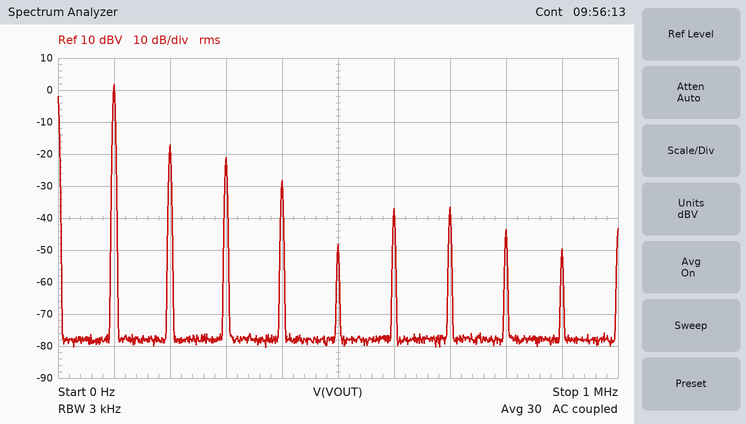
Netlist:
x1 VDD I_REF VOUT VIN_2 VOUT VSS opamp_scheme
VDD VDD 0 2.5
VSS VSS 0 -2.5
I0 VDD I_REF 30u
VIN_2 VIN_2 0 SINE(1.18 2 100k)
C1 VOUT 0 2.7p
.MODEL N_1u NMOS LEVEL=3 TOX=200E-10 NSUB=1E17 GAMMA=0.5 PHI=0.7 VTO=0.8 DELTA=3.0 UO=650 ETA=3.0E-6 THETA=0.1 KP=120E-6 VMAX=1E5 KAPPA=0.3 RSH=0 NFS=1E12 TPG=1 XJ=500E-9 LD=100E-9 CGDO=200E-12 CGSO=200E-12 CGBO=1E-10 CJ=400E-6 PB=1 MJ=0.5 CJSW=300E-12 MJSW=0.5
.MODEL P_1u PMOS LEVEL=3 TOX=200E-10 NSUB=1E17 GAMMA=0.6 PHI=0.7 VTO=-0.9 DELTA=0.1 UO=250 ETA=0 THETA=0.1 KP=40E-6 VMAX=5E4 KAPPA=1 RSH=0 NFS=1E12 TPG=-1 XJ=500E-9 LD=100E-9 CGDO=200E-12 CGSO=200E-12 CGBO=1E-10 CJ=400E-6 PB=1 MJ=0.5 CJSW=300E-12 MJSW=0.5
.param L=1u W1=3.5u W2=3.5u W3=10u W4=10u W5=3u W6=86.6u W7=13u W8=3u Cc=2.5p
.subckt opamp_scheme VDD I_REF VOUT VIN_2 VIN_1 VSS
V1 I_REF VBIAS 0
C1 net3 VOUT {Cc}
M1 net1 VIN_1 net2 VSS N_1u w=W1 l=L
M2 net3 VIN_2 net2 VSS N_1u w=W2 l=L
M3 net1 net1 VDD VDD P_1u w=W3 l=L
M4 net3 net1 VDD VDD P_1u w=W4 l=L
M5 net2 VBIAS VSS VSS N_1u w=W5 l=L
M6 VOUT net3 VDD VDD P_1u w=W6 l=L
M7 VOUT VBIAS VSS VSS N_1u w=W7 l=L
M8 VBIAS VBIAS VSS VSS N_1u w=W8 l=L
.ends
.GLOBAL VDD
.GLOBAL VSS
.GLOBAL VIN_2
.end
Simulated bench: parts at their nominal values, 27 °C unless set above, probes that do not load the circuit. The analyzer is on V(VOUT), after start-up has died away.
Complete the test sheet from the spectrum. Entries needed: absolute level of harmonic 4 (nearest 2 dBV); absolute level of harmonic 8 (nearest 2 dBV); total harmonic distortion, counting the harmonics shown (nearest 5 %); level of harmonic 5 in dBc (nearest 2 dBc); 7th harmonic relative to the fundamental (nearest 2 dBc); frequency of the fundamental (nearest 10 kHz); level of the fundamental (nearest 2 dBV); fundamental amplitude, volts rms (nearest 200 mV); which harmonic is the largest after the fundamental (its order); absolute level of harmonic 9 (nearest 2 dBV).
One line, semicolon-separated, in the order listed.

-28 dBV; -44 dBV; 15 %; -50 dBc; -38 dBc; 100 kHz; 2 dBV; 1.2 V; 2; -50 dBV
